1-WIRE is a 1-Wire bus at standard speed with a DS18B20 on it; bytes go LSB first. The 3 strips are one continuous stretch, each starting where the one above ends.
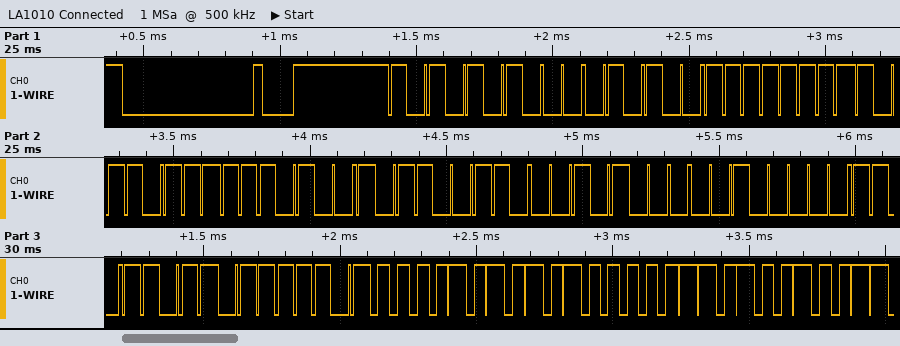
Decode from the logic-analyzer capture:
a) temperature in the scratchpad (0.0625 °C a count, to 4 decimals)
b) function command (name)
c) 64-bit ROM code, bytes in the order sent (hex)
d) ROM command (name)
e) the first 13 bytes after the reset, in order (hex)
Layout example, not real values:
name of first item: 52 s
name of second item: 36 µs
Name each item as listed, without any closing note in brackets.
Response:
temperature in the scratchpad: 85.0000 °C
function command: Read Scratchpad
64-bit ROM code, bytes in the order sent: 28 FF ED 97 66 14 04 DB
ROM command: Match ROM
the first 13 bytes after the reset, in order: 55 28 FF ED 97 66 14 04 DB BE 50 05 4B
